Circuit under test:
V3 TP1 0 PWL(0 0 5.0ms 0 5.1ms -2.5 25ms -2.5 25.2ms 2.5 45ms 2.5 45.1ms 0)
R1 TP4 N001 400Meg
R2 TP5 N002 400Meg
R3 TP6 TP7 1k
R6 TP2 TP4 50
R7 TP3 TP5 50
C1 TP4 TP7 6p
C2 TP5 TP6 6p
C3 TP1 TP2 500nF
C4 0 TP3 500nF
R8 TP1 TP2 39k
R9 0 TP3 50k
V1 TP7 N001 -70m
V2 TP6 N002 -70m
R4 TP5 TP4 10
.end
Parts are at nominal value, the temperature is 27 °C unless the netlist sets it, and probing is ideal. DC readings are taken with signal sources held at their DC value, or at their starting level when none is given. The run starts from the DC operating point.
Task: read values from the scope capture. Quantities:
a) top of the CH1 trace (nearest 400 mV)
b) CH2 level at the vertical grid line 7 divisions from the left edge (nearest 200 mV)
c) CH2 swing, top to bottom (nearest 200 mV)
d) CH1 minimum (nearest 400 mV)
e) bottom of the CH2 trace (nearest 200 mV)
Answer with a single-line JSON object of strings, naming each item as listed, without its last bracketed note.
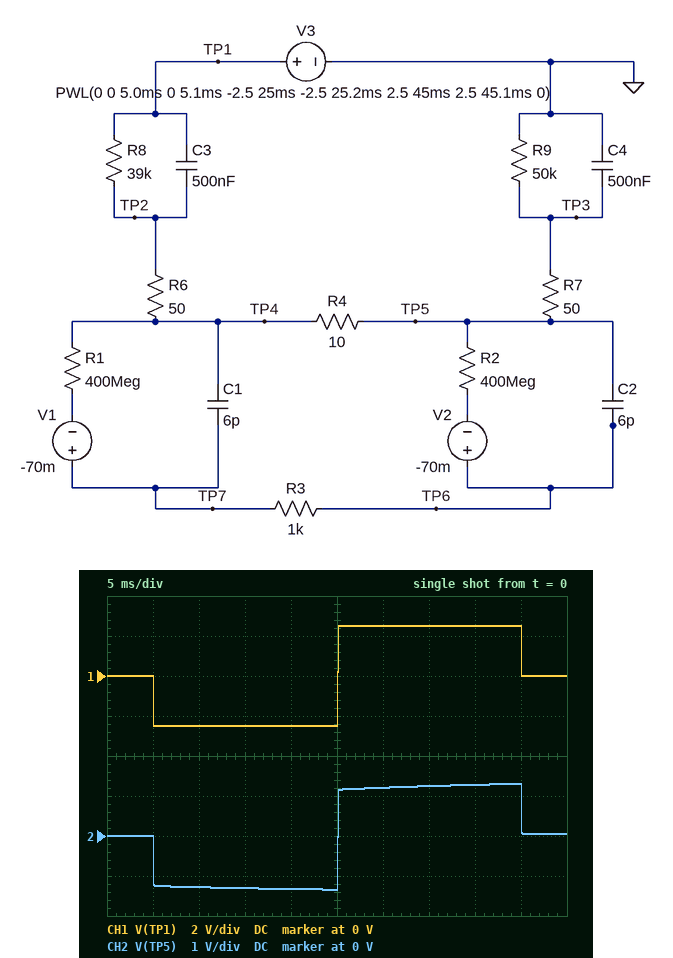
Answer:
{"top of the CH1 trace": "2.4 V", "CH2 level at the vertical grid line 7 divisions from the left edge": "1.2 V", "CH2 swing, top to bottom": "2.6 V", "CH1 minimum": "-2.4 V", "bottom of the CH2 trace": "-1.4 V"}
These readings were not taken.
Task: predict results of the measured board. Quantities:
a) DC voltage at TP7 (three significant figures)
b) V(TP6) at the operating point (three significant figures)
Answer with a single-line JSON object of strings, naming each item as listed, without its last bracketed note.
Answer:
{"DC voltage at TP7": "-70.0 mV", "V(TP6) at the operating point": "-70.0 mV"}
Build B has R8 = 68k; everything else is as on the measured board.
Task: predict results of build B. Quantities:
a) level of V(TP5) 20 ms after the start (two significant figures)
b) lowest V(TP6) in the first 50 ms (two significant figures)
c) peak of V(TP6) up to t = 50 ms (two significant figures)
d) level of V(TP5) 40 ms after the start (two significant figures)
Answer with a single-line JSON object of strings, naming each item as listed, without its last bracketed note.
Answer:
{"level of V(TP5) 20 ms after the start": "-1.2 V", "lowest V(TP6) in the first 50 ms": "-1.3 V", "peak of V(TP6) up to t = 50 ms": "1.3 V", "level of V(TP5) 40 ms after the start": "1.2 V"}
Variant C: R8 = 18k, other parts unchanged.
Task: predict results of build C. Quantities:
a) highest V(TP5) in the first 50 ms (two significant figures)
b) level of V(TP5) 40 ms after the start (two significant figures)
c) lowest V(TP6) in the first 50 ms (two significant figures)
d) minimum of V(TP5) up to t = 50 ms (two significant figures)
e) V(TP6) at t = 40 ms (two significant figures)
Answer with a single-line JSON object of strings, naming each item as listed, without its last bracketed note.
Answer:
{"highest V(TP5) in the first 50 ms": "1.6 V", "level of V(TP5) 40 ms after the start": "1.5 V", "lowest V(TP6) in the first 50 ms": "-1.8 V", "minimum of V(TP5) up to t = 50 ms": "-1.7 V", "V(TP6) at t = 40 ms": "1.4 V"}
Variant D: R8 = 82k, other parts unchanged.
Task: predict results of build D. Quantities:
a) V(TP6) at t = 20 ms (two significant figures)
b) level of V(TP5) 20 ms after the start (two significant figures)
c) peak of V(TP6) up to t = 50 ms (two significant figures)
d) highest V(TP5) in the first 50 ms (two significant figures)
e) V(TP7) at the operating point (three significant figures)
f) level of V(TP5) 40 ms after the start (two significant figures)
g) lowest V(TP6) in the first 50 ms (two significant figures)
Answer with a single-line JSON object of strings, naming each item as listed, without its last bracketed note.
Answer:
{"V(TP6) at t = 20 ms": "-1.2 V", "level of V(TP5) 20 ms after the start": "-1.1 V", "peak of V(TP6) up to t = 50 ms": "1.3 V", "highest V(TP5) in the first 50 ms": "1.4 V", "V(TP7) at the operating point": "-70.0 mV", "level of V(TP5) 40 ms after the start": "1.2 V", "lowest V(TP6) in the first 50 ms": "-1.3 V"}
